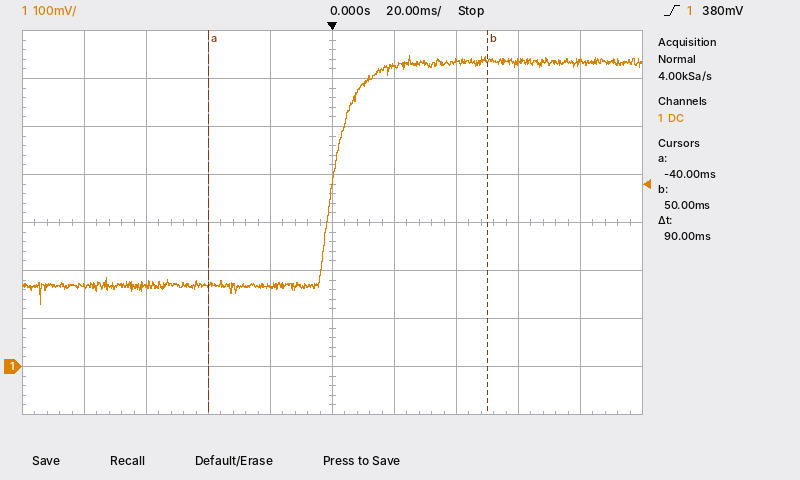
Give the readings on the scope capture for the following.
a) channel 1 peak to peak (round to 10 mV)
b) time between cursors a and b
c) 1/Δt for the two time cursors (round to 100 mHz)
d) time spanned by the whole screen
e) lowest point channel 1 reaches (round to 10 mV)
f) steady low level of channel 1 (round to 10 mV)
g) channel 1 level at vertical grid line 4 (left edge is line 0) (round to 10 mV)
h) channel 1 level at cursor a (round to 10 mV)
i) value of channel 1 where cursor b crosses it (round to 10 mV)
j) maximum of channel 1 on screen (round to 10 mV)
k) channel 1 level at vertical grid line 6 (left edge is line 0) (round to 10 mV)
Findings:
520 mV
90 ms
11.1 Hz
200 ms
130 mV
170 mV
170 mV
170 mV
640 mV
650 mV
630 mV
